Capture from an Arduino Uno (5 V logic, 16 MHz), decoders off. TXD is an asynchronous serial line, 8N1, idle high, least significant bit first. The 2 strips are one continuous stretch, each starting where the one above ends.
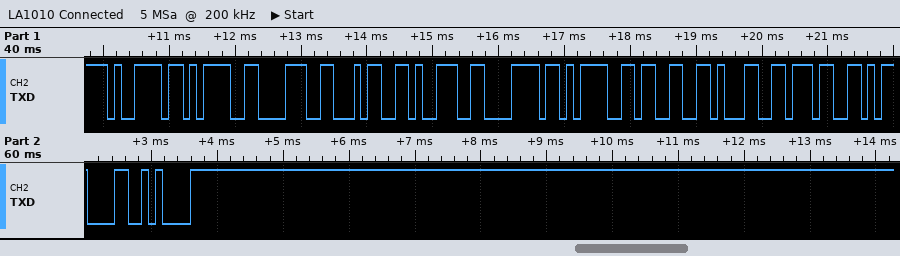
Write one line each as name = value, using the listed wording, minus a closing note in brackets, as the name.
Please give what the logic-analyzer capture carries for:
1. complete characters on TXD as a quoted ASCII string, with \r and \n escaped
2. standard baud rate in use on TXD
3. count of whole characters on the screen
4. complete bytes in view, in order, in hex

complete characters on TXD as a quoted ASCII string, with \r and \n escaped = "y=849x=317\r\n"
standard baud rate in use on TXD = 9600 baud
count of whole characters on the screen = 12
complete bytes in view, in order, in hex = 79 3D 38 34 39 78 3D 33 31 37 0D 0A
